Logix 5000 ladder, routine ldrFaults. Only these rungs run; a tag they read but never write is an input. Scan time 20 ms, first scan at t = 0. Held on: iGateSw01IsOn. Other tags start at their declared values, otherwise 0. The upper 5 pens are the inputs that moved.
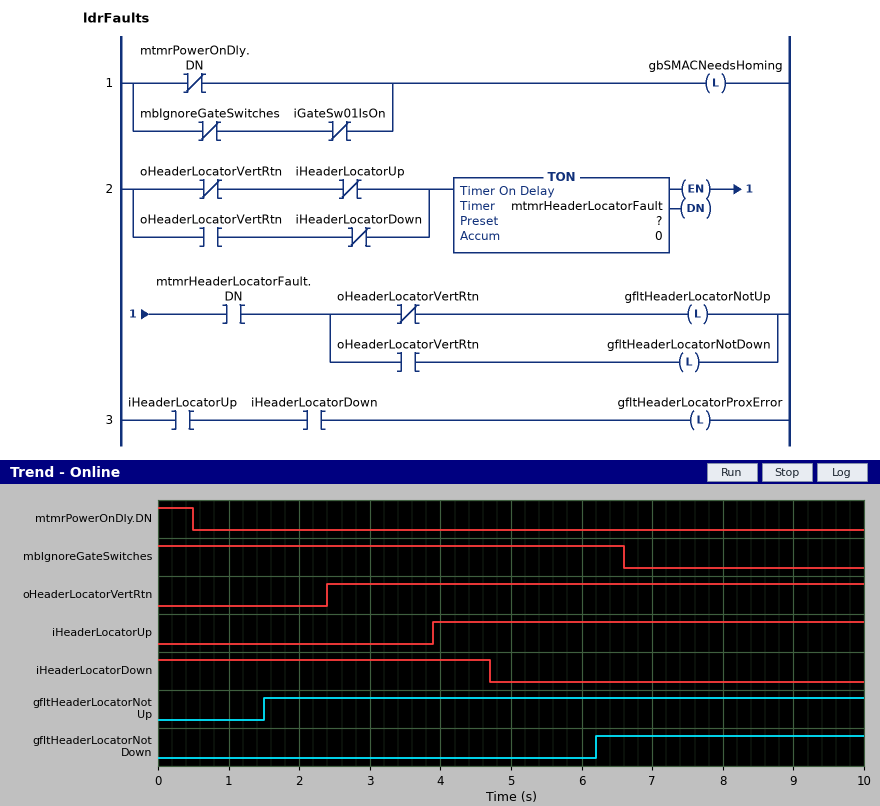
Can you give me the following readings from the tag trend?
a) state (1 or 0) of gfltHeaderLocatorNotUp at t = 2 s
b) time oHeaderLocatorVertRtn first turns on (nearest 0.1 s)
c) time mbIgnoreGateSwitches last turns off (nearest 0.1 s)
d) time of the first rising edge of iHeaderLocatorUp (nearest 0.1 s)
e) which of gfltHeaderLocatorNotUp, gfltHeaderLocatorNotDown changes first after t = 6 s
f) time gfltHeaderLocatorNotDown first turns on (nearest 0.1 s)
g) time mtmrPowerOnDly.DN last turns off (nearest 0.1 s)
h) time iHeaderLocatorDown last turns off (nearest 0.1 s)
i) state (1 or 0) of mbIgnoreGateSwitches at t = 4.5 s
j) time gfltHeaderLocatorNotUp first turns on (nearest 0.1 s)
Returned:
1
2.4 s
6.6 s
3.9 s
gfltHeaderLocatorNotDown
6.2 s
0.5 s
4.7 s
1
1.5 s
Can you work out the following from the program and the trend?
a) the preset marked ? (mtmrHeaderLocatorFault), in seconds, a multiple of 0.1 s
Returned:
1.5 s
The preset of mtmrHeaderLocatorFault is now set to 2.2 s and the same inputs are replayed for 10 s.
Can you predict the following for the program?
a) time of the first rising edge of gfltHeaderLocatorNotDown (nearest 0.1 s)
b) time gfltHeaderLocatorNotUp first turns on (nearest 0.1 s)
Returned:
6.9 s
2.2 s
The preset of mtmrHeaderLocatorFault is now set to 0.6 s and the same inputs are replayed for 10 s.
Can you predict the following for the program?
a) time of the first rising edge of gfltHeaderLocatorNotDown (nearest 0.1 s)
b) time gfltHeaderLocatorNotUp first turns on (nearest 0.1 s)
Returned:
5.3 s
0.6 s
